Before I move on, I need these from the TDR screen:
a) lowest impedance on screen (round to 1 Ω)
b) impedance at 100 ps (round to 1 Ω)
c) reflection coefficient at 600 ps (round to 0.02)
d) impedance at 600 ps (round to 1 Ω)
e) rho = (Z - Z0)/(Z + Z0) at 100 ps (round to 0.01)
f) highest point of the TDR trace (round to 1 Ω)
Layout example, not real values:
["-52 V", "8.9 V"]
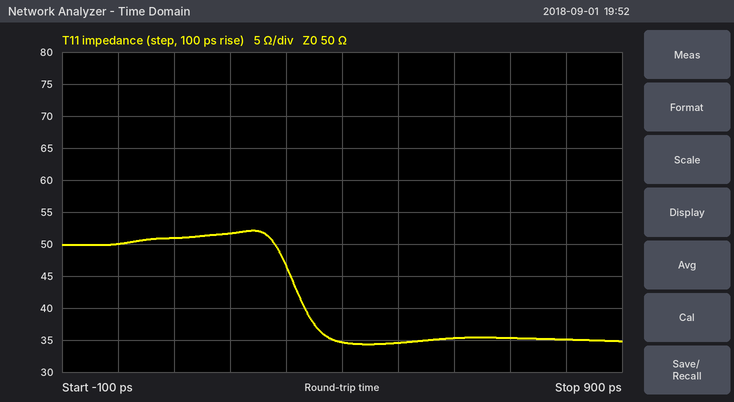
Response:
["34 Ω", "51 Ω", "-0.18", "35 Ω", "+0.01", "52 Ω"]
